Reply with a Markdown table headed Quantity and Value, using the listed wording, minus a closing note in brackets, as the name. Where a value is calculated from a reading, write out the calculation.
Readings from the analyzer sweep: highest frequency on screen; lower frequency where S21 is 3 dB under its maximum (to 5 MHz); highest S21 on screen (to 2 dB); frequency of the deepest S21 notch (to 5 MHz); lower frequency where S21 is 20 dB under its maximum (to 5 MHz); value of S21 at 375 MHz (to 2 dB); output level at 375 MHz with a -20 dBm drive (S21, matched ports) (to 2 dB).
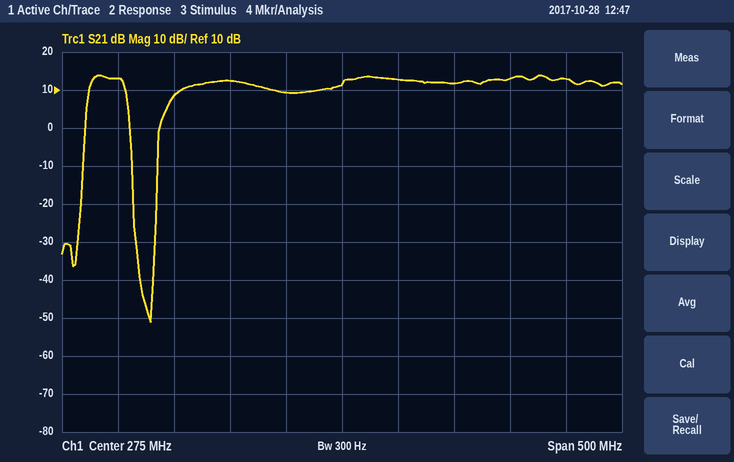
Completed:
| Quantity | Value |
|---|---|
| highest frequency on screen | 525 MHz |
| lower frequency where S21 is 3 dB under its maximum | 50 MHz |
| highest S21 on screen | 14 dB |
| frequency of the deepest S21 notch | 105 MHz |
| lower frequency where S21 is 20 dB under its maximum | 45 MHz |
| value of S21 at 375 MHz | 12 dB |
| output level at 375 MHz with a -20 dBm drive (S21, matched ports) | -20 dBm + (12 dB) = -8 dBm |
